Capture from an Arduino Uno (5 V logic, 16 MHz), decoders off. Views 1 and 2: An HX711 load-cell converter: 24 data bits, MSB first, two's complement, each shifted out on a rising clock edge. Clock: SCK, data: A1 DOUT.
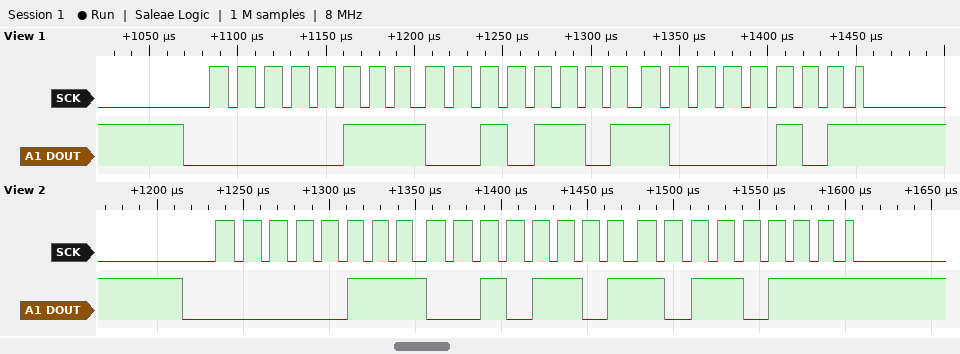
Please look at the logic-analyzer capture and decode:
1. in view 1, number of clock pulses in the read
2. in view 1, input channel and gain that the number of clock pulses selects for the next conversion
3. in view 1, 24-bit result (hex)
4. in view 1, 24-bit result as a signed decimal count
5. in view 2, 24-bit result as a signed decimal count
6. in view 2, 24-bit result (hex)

25
channel A, gain 128
0x072D85
470405
470455
0x072DB7
